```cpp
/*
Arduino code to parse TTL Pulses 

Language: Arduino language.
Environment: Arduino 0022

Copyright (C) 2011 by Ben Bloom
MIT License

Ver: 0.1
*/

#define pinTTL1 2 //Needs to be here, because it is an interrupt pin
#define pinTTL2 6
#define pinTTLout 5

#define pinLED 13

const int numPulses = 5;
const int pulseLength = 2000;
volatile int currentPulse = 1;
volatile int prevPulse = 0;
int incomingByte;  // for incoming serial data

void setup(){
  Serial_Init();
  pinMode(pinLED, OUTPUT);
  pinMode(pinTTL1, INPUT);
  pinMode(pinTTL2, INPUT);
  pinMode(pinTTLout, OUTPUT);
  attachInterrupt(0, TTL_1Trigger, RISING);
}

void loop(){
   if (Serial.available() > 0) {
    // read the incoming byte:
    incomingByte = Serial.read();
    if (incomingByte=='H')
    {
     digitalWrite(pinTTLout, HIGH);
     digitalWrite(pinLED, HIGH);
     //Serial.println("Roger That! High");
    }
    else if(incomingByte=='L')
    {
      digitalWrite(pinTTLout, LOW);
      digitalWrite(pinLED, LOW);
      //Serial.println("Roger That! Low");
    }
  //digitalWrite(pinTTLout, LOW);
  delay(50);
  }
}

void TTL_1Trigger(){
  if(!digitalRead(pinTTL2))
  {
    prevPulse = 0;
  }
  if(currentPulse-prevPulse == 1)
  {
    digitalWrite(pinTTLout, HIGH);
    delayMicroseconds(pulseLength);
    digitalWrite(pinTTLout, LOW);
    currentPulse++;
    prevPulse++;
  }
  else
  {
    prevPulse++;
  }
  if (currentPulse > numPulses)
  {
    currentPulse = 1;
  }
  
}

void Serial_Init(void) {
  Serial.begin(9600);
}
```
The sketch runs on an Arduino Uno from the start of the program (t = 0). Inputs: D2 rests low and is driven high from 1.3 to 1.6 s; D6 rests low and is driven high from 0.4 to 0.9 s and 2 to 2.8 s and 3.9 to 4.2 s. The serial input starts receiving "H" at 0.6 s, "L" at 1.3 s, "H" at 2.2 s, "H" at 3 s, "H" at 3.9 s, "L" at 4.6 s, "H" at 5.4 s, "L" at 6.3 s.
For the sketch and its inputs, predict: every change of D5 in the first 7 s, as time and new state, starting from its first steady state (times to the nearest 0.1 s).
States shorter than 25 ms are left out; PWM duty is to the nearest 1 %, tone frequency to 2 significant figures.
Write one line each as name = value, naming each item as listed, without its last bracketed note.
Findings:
every change of D5 in the first 7 s, as time and new state, starting from its first steady state = 0 s low; 0.6 s high; 1.3 s low; 2.2 s high; 4.6 s low; 5.4 s high; 6.3 s low
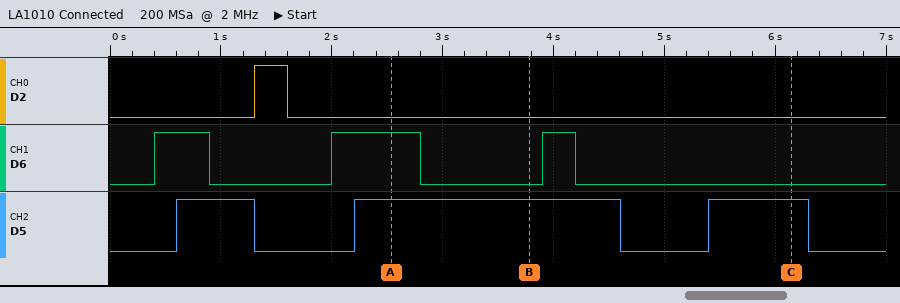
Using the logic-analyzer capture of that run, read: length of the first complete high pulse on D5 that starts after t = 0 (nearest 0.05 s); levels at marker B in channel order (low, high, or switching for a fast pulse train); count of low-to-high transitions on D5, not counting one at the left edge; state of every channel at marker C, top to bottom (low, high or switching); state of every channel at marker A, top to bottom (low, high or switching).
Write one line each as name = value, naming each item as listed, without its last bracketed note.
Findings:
length of the first complete high pulse on D5 that starts after t = 0 = 0.70 s
levels at marker B in channel order = D2 low, D6 low, D5 high
count of low-to-high transitions on D5, not counting one at the left edge = 3
state of every channel at marker C, top to bottom = D2 low, D6 low, D5 high
state of every channel at marker A, top to bottom = D2 low, D6 high, D5 high
